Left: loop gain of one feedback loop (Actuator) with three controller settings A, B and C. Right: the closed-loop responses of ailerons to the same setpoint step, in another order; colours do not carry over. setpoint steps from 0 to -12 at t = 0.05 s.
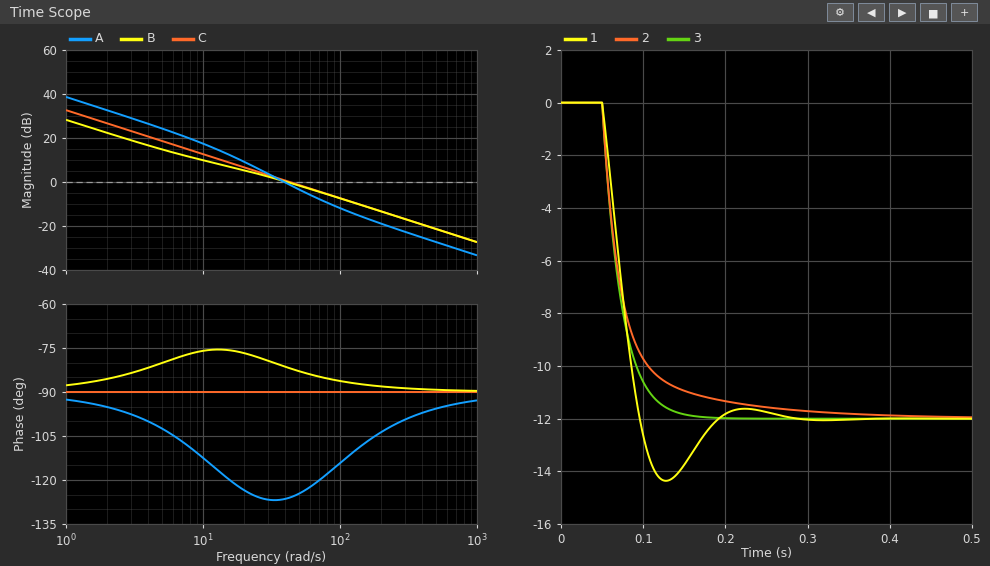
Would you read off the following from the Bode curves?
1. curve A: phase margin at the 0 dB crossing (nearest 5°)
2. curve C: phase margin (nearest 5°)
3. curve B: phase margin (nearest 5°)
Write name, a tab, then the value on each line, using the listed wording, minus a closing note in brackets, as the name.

curve A: phase margin at the 0 dB crossing	55°
curve C: phase margin	90°
curve B: phase margin	100°
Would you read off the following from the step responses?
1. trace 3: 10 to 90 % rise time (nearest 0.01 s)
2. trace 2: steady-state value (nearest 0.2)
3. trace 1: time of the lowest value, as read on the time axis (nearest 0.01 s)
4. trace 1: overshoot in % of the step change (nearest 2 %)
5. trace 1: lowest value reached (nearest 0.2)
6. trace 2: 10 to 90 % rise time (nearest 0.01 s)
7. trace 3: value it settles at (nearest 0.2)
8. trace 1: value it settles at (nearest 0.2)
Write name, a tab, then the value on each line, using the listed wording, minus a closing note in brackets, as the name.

trace 3: 10 to 90 % rise time	0.05 s
trace 2: steady-state value	-12.0
trace 1: time of the lowest value, as read on the time axis	0.13 s
trace 1: overshoot in % of the step change	20 %
trace 1: lowest value reached	-14.4
trace 2: 10 to 90 % rise time	0.09 s
trace 3: value it settles at	-12.0
trace 1: value it settles at	-12.0
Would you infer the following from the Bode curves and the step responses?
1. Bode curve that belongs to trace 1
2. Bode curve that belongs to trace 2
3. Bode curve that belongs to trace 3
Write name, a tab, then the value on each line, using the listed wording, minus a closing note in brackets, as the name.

Bode curve that belongs to trace 1	A
Bode curve that belongs to trace 2	B
Bode curve that belongs to trace 3	C
